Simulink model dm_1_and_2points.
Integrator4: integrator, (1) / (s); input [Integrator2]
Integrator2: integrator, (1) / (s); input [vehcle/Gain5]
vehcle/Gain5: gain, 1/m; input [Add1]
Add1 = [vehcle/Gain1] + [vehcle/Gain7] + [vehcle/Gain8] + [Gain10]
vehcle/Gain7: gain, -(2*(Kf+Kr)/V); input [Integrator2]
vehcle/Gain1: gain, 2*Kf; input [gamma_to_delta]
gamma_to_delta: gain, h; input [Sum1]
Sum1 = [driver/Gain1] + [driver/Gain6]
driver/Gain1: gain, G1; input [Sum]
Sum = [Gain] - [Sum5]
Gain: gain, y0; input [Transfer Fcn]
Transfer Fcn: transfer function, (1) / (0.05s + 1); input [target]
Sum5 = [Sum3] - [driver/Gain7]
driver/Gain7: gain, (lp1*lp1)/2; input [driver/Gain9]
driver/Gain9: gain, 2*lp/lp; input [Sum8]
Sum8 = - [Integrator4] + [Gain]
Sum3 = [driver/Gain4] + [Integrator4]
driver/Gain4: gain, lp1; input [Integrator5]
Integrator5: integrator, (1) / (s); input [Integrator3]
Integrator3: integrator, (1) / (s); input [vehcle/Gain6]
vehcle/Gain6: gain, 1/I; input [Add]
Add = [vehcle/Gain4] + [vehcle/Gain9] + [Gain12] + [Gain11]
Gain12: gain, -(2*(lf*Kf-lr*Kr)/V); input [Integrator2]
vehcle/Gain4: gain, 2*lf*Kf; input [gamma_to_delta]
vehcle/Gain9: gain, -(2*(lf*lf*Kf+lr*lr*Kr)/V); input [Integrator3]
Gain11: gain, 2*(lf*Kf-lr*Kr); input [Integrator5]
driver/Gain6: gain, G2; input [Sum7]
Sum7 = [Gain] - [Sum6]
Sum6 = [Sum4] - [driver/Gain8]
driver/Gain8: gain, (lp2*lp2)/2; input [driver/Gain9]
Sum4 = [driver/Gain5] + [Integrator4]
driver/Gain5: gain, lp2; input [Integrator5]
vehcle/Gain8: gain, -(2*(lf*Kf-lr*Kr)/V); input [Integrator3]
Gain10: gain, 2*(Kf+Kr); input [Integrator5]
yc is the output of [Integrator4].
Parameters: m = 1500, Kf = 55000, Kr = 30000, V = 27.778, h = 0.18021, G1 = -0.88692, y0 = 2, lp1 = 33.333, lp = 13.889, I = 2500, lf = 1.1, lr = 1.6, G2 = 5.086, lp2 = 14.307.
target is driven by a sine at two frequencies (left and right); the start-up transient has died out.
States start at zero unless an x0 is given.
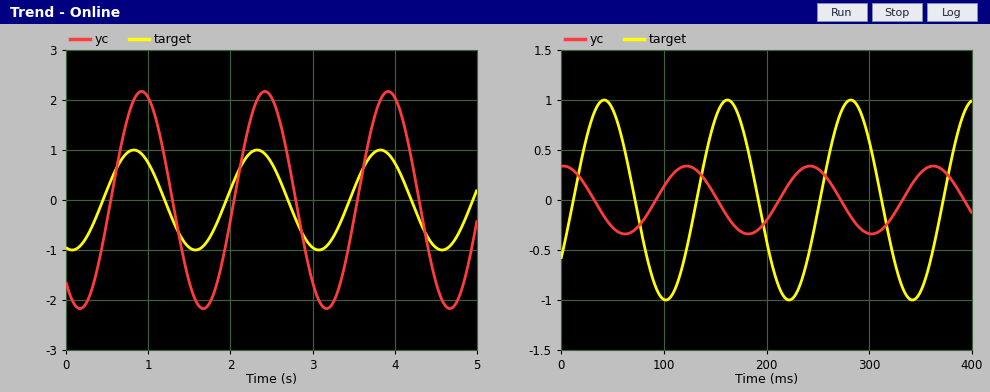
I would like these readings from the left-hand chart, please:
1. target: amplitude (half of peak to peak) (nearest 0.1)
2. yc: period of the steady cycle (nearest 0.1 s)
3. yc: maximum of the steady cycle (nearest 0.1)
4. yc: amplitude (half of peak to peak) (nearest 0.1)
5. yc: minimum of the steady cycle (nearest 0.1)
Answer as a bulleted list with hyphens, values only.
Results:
- 1.0
- 1.5 s
- 2.2
- 2.2
- -2.2
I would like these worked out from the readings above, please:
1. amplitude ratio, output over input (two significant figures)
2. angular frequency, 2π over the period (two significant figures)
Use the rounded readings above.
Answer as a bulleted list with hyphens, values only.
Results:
- 2.2
- 4.2 rad/s
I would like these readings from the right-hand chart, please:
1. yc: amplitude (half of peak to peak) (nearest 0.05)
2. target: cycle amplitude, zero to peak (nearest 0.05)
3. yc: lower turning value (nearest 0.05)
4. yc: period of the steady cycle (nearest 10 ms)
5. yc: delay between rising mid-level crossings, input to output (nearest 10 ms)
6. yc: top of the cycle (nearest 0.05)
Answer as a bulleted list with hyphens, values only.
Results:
- 0.35
- 1.00
- -0.35
- 120 ms
- 80 ms
- 0.35
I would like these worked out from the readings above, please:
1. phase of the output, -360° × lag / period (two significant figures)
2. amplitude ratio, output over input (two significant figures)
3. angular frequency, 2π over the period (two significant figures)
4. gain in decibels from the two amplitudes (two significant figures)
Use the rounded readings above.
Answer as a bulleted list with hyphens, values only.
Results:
- -240°
- 0.35
- 0.052 rad/ms
- -9.1 dB
